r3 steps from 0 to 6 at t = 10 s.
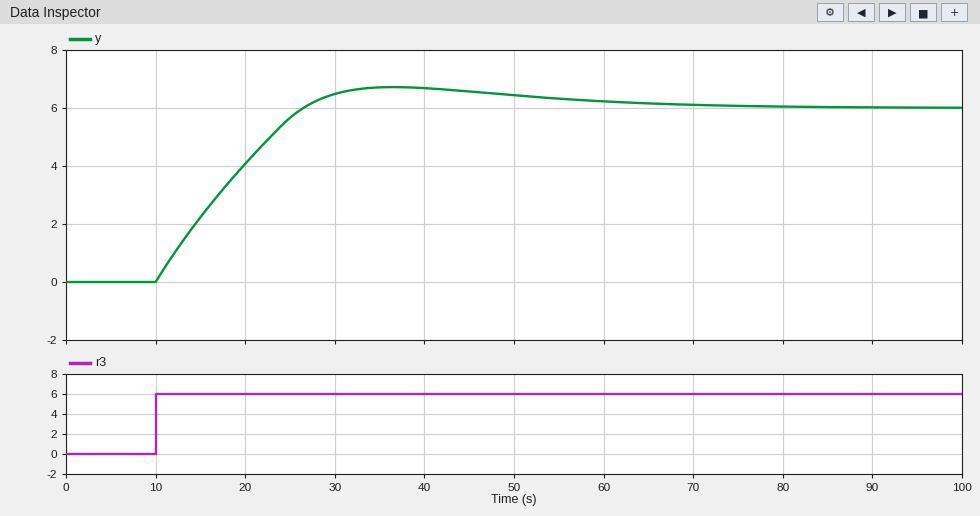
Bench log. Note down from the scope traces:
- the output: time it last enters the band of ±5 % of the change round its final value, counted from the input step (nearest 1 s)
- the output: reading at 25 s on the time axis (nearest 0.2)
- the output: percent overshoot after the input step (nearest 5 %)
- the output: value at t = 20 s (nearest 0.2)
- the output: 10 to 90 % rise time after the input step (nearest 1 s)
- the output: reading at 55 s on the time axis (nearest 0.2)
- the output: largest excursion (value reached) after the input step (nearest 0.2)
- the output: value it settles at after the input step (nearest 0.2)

46 s
5.6
10 %
4.0
13 s
6.4
6.8
6.0
